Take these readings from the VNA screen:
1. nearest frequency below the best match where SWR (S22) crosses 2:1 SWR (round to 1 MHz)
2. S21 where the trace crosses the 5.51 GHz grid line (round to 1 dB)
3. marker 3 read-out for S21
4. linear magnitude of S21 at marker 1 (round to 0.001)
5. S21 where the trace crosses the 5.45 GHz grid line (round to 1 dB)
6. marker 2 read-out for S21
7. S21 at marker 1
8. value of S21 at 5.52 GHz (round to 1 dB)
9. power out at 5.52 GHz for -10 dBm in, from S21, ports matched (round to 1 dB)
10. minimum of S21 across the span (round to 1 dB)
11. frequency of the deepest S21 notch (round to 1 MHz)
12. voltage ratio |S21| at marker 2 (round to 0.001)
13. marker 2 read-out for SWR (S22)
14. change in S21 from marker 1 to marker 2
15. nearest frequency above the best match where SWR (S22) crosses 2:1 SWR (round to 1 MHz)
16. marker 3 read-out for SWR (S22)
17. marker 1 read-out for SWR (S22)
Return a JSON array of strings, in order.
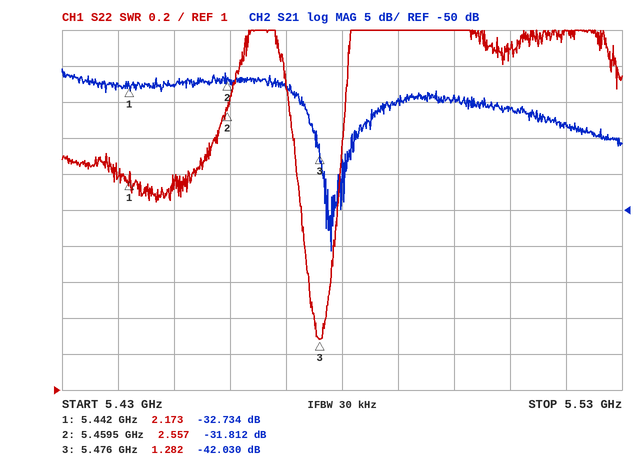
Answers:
["5.473 GHz", "-36 dB", "-42.030 dB", "0.023", "-33 dB", "-31.812 dB", "-32.734 dB", "-38 dB", "-48 dBm", "-56 dB", "5.478 GHz", "0.026", "2.557", "0.922 dB", "5.479 GHz", "1.282", "2.173"]
